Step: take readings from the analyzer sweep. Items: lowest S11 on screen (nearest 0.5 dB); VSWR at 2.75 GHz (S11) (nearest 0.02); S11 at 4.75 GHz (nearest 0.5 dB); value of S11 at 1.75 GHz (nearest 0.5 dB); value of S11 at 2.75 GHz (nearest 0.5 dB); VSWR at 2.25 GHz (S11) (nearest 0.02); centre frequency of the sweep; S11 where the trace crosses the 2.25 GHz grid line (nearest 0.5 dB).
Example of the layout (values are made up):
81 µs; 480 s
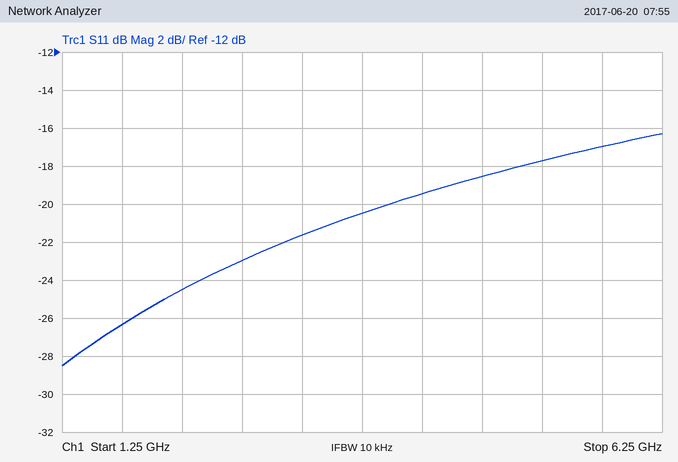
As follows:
-28.5 dB; 1.16; -18.5 dB; -26.5 dB; -23.0 dB; 1.12; 3.75 GHz; -24.5 dB
